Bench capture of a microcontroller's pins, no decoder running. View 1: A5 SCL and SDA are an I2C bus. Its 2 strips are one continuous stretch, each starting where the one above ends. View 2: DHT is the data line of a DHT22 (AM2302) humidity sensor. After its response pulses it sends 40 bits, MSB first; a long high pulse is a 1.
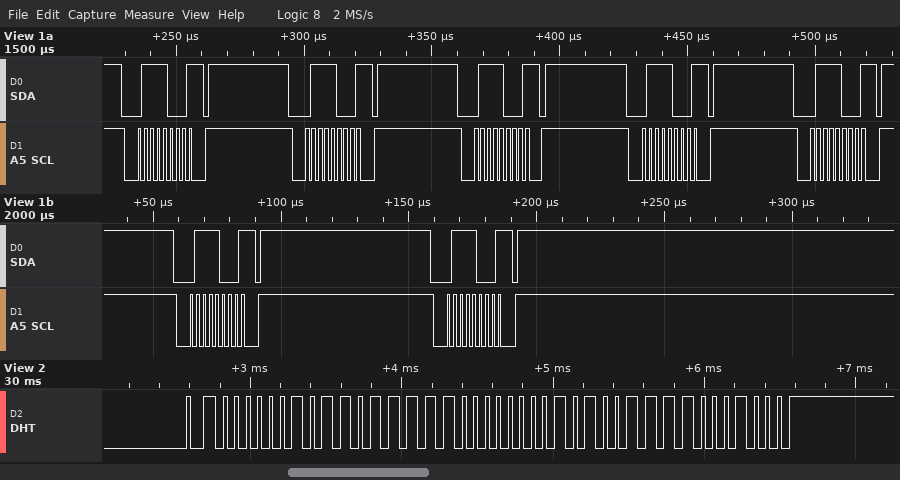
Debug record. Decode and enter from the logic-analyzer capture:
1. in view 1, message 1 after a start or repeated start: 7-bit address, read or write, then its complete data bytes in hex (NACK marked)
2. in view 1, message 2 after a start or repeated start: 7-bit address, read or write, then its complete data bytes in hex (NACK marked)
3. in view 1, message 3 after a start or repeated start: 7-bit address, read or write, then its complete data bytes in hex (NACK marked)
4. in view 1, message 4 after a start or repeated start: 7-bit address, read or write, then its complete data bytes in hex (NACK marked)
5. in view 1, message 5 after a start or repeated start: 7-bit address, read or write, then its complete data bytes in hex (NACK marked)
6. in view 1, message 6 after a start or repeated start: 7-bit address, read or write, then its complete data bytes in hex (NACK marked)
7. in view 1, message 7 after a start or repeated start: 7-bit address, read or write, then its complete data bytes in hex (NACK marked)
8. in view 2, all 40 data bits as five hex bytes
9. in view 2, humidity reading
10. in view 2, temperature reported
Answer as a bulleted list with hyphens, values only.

- 0x3C write NACK
- 0x3C write NACK
- 0x3C write NACK
- 0x3C write NACK
- 0x3C write NACK
- 0x3C write NACK
- 0x3C write NACK
- 02 DF 00 A7 88
- 73.5 %
- 16.7 °C
